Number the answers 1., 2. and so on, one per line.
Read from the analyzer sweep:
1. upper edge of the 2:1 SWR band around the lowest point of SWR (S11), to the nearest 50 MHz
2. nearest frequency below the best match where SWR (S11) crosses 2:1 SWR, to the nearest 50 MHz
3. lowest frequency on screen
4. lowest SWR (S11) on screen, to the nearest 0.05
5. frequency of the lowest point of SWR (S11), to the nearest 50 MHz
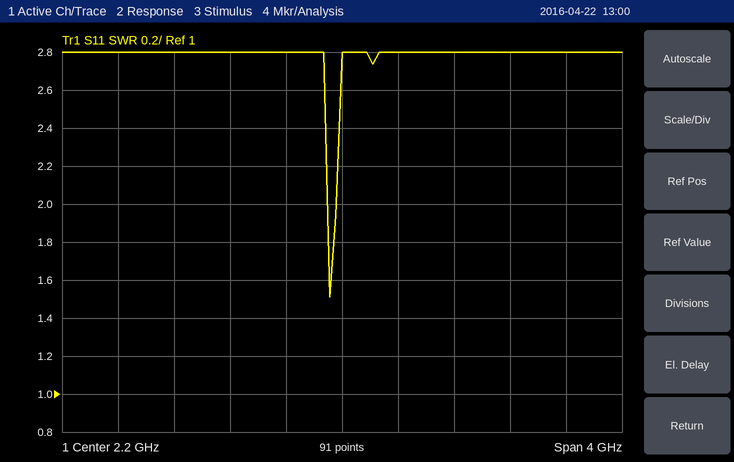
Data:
1. 2.15 GHz
2. 2.10 GHz
3. 200 MHz
4. 1.50
5. 2.10 GHz
